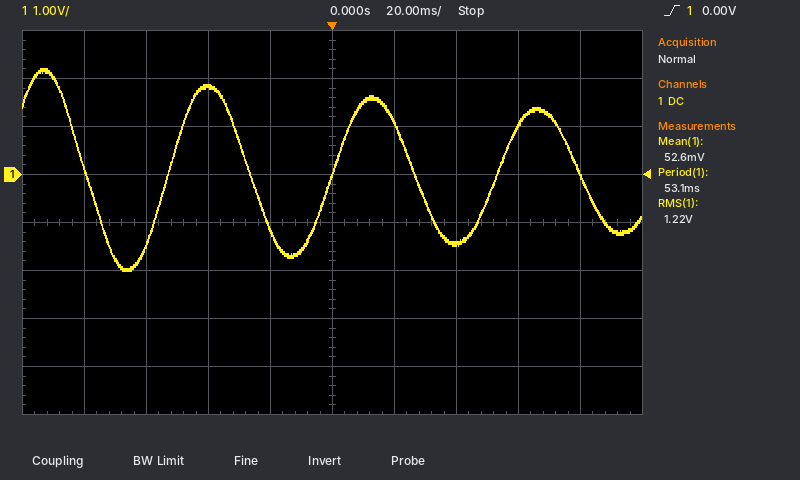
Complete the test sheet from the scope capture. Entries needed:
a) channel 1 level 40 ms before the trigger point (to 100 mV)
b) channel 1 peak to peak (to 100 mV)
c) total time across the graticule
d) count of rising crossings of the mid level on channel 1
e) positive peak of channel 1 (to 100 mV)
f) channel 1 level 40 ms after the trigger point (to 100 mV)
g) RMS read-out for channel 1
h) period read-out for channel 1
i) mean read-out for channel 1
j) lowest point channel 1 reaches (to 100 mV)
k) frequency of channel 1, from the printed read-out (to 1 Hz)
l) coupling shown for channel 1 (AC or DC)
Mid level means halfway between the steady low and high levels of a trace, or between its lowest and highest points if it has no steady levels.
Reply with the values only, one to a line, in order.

1.8 V
4.2 V
200 ms
3
2.2 V
-1.4 V
1.22 V
53.1 ms
52.6 mV
-2.0 V
19 Hz
DC
